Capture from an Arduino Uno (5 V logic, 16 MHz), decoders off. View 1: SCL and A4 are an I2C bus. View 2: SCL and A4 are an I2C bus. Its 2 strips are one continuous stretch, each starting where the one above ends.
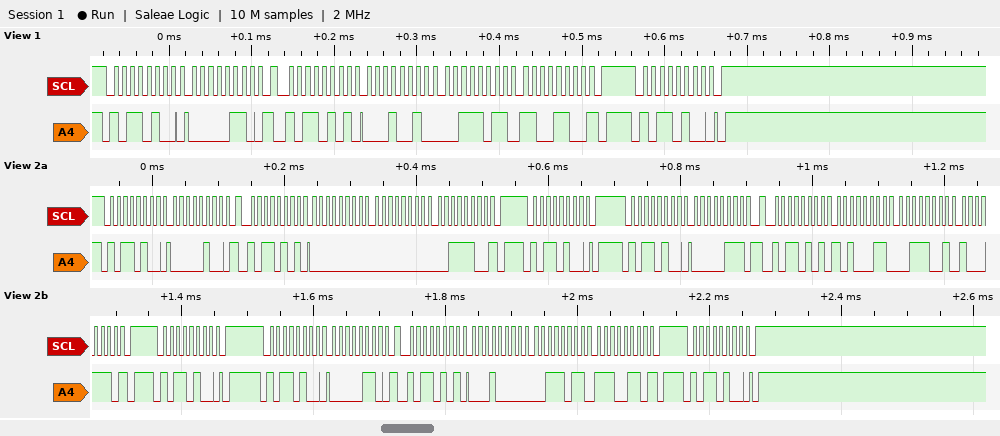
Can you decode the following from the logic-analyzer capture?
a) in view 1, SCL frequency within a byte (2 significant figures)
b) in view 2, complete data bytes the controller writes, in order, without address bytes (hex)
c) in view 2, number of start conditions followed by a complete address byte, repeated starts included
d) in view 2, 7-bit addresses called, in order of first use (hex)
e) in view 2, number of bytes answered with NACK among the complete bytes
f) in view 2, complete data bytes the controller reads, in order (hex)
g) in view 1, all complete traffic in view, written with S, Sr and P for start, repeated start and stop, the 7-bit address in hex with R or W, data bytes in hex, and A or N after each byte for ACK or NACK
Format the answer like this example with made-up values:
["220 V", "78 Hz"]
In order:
["100 kHz", "04 07 06", "9", "0x5A", "3", "00 00 3C A3 39 8E 10 3B E6", "S 5AW A 06 A Sr 5AR A 12 A 3B A CC N P S 5AW A P"]
